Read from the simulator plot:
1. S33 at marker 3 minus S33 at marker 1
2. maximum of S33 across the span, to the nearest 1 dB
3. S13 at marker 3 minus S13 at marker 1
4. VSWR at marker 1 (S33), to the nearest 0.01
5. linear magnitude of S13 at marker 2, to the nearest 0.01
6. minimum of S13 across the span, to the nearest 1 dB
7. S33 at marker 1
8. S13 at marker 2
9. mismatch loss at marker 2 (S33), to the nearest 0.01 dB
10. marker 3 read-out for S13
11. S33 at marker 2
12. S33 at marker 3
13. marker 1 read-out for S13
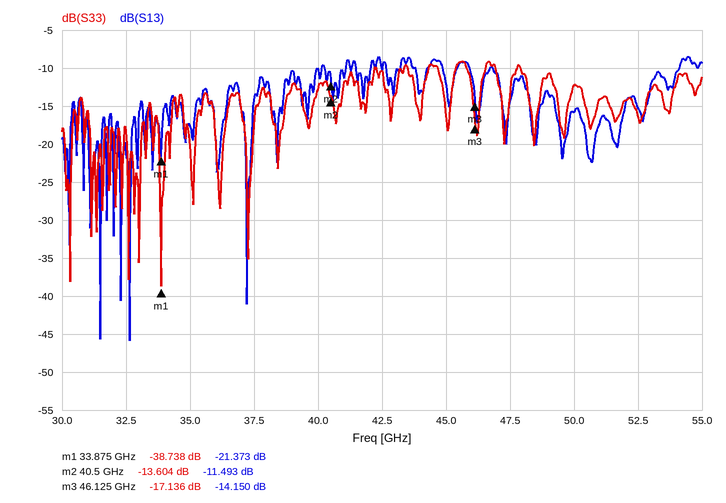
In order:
21.602 dB
-9 dB
7.223 dB
1.02
0.27
-46 dB
-38.738 dB
-11.493 dB
0.19 dB
-14.150 dB
-13.604 dB
-17.136 dB
-21.373 dB
